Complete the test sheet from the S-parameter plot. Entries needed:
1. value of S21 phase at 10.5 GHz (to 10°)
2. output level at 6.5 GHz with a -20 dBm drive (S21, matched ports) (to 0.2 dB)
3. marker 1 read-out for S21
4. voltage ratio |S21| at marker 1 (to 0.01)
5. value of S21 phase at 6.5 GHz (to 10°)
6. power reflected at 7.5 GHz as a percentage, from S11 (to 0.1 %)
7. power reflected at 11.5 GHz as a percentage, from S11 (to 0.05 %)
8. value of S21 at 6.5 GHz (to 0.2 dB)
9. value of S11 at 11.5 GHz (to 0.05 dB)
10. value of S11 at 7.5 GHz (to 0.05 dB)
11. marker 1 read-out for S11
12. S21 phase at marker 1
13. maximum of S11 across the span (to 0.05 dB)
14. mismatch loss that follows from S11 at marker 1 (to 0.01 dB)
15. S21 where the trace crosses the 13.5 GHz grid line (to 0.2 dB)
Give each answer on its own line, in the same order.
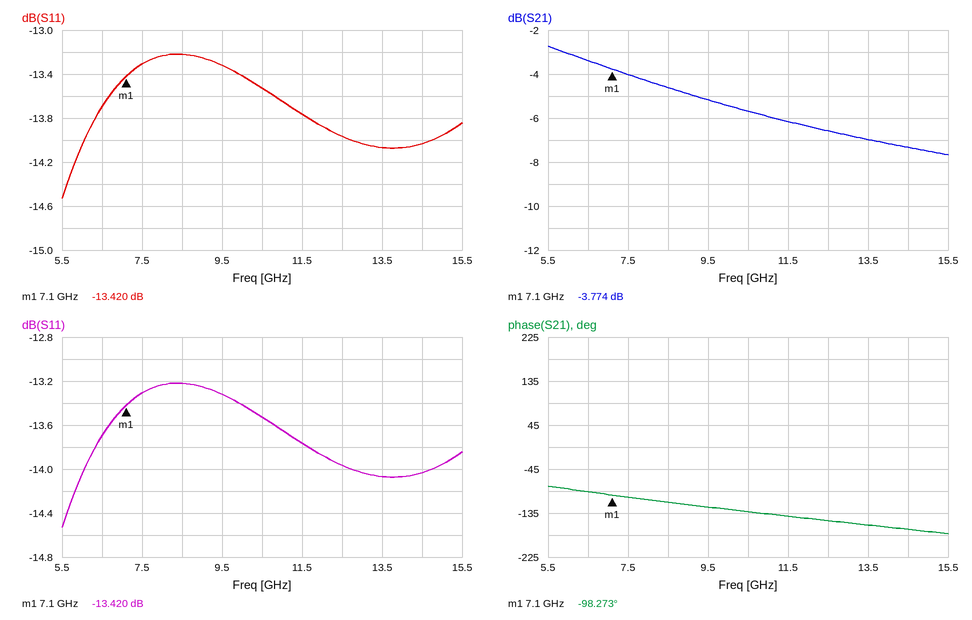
-130°
-23.4 dBm
-3.774 dB
0.65
-90°
4.7 %
4.20 %
-3.4 dB
-13.75 dB
-13.30 dB
-13.420 dB
-98.273°
-13.20 dB
0.20 dB
-7.0 dB
